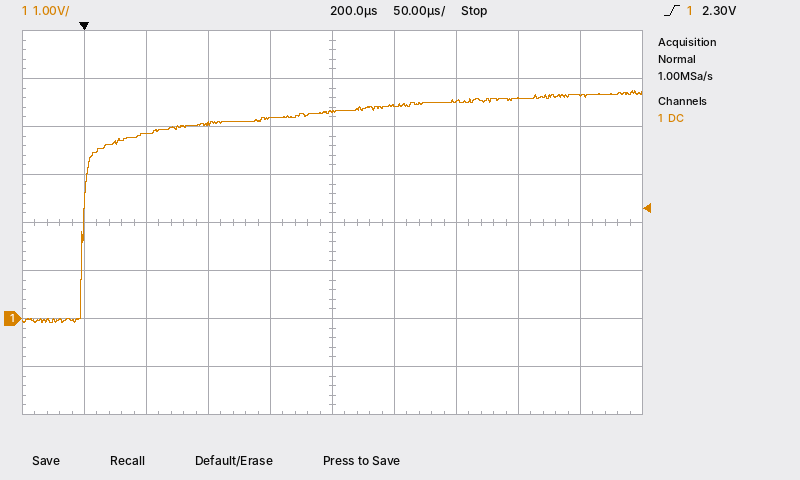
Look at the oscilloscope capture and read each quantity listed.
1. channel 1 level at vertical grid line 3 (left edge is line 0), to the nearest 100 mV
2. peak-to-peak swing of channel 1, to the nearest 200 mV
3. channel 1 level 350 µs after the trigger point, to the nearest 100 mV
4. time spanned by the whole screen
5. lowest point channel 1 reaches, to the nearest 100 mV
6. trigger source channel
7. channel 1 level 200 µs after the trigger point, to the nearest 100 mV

4.1 V
4.8 V
4.6 V
500 µs
-100 mV
channel 1
4.3 V
